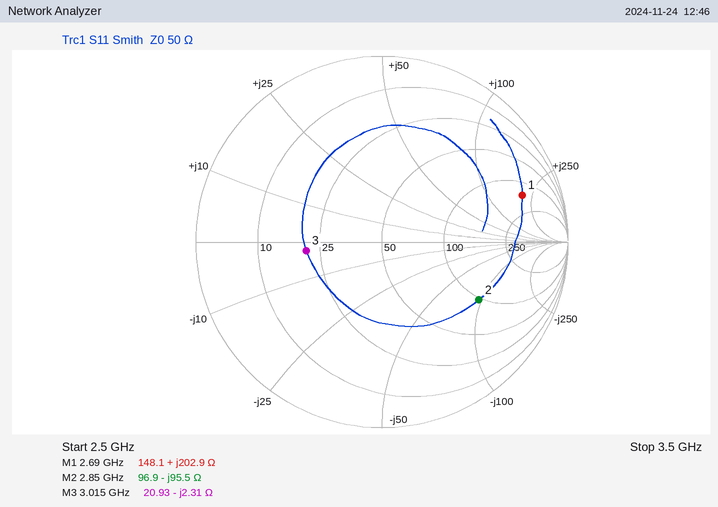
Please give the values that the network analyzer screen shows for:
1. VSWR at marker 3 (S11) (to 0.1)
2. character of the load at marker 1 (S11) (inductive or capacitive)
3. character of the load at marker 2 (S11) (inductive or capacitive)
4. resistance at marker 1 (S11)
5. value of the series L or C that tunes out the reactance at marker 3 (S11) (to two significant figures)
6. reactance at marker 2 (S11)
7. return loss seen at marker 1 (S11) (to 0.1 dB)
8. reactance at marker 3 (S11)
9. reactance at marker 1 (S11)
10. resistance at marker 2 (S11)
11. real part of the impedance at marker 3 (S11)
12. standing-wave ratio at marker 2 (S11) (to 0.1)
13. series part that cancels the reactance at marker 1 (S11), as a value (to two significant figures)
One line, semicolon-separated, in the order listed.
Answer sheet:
2.4; inductive; capacitive; 148.1 Ω; 120 pH; -95.5 Ω; 2.0 dB; -2.31 Ω; +202.9 Ω; 96.9 Ω; 20.93 Ω; 4.1; 290 fF
